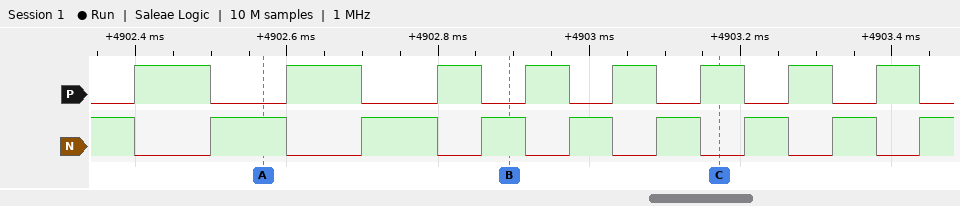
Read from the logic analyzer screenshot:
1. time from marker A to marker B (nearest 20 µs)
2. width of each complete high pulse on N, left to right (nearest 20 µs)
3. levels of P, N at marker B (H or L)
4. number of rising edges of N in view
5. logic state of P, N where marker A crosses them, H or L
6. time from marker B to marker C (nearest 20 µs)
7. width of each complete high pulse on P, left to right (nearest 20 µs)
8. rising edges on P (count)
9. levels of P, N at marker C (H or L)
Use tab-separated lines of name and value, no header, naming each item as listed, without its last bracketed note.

time from marker A to marker B	320 µs
width of each complete high pulse on N, left to right	100 µs, 100 µs, 60 µs, 60 µs, 60 µs, 60 µs, 60 µs
levels of P, N at marker B	P=L, N=H
number of rising edges of N in view	8
logic state of P, N where marker A crosses them, H or L	P=L, N=H
time from marker B to marker C	280 µs
width of each complete high pulse on P, left to right	100 µs, 100 µs, 60 µs, 60 µs, 60 µs, 60 µs, 60 µs, 60 µs
rising edges on P	8
levels of P, N at marker C	P=H, N=L
